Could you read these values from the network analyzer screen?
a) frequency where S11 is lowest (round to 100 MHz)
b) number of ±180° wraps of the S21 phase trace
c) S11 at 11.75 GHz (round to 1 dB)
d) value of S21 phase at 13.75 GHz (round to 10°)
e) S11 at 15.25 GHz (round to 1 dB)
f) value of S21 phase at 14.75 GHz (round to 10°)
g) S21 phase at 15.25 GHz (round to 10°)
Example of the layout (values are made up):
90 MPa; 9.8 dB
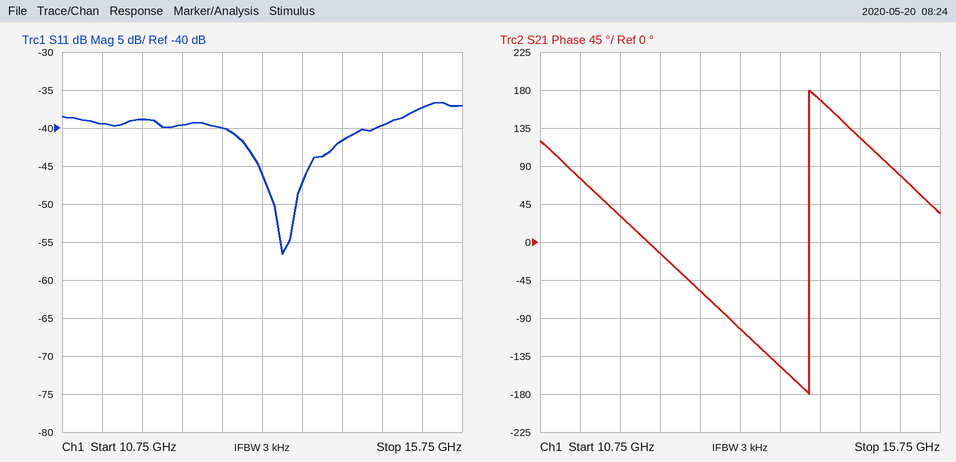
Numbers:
13.5 GHz; 1; -39 dB; -150°; -37 dB; 120°; 80°
